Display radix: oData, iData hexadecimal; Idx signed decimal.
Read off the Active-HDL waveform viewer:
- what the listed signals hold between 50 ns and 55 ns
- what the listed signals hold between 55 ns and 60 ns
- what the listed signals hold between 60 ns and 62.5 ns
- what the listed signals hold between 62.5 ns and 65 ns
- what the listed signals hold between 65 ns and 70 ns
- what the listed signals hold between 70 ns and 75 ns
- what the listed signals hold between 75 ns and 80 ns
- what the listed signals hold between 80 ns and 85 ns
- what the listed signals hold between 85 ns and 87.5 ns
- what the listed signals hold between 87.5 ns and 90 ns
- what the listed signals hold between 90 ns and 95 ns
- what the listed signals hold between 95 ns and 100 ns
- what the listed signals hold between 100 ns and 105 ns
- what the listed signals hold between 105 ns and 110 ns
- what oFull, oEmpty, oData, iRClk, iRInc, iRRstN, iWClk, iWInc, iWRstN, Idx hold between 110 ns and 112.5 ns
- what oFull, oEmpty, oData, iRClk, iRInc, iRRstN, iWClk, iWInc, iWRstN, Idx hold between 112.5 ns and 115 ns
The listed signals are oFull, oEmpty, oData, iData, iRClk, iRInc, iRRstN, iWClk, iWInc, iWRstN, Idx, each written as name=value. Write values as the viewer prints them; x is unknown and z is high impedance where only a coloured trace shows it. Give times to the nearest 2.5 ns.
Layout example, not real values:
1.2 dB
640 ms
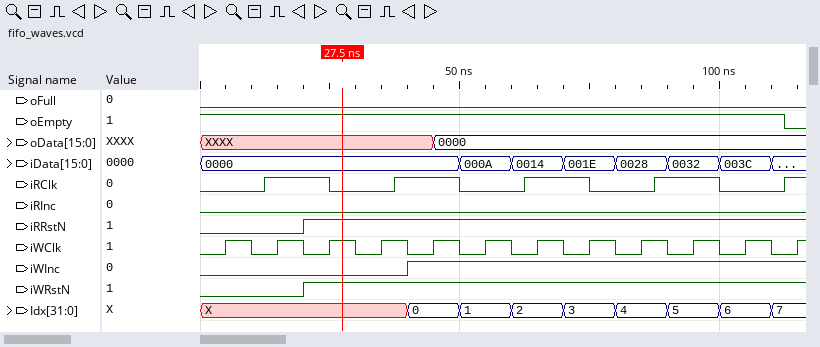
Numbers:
oFull=0, oEmpty=1, oData=0000, iData=000A, iRClk=0, iRInc=0, iRRstN=1, iWClk=0, iWInc=1, iWRstN=1, Idx=1
oFull=0, oEmpty=1, oData=0000, iData=000A, iRClk=0, iRInc=0, iRRstN=1, iWClk=1, iWInc=1, iWRstN=1, Idx=1
oFull=0, oEmpty=1, oData=0000, iData=0014, iRClk=0, iRInc=0, iRRstN=1, iWClk=0, iWInc=1, iWRstN=1, Idx=2
oFull=0, oEmpty=1, oData=0000, iData=0014, iRClk=1, iRInc=0, iRRstN=1, iWClk=0, iWInc=1, iWRstN=1, Idx=2
oFull=0, oEmpty=1, oData=0000, iData=0014, iRClk=1, iRInc=0, iRRstN=1, iWClk=1, iWInc=1, iWRstN=1, Idx=2
oFull=0, oEmpty=1, oData=0000, iData=001E, iRClk=1, iRInc=0, iRRstN=1, iWClk=0, iWInc=1, iWRstN=1, Idx=3
oFull=0, oEmpty=1, oData=0000, iData=001E, iRClk=0, iRInc=0, iRRstN=1, iWClk=1, iWInc=1, iWRstN=1, Idx=3
oFull=0, oEmpty=1, oData=0000, iData=0028, iRClk=0, iRInc=0, iRRstN=1, iWClk=0, iWInc=1, iWRstN=1, Idx=4
oFull=0, oEmpty=1, oData=0000, iData=0028, iRClk=0, iRInc=0, iRRstN=1, iWClk=1, iWInc=1, iWRstN=1, Idx=4
oFull=0, oEmpty=1, oData=0000, iData=0028, iRClk=1, iRInc=0, iRRstN=1, iWClk=1, iWInc=1, iWRstN=1, Idx=4
oFull=0, oEmpty=1, oData=0000, iData=0032, iRClk=1, iRInc=0, iRRstN=1, iWClk=0, iWInc=1, iWRstN=1, Idx=5
oFull=0, oEmpty=1, oData=0000, iData=0032, iRClk=1, iRInc=0, iRRstN=1, iWClk=1, iWInc=1, iWRstN=1, Idx=5
oFull=0, oEmpty=1, oData=0000, iData=003C, iRClk=0, iRInc=0, iRRstN=1, iWClk=0, iWInc=1, iWRstN=1, Idx=6
oFull=0, oEmpty=1, oData=0000, iData=003C, iRClk=0, iRInc=0, iRRstN=1, iWClk=1, iWInc=1, iWRstN=1, Idx=6
oFull=0, oEmpty=1, oData=0000, iRClk=0, iRInc=0, iRRstN=1, iWClk=0, iWInc=1, iWRstN=1, Idx=7
oFull=0, oEmpty=0, oData=0000, iRClk=1, iRInc=0, iRRstN=1, iWClk=0, iWInc=1, iWRstN=1, Idx=7
